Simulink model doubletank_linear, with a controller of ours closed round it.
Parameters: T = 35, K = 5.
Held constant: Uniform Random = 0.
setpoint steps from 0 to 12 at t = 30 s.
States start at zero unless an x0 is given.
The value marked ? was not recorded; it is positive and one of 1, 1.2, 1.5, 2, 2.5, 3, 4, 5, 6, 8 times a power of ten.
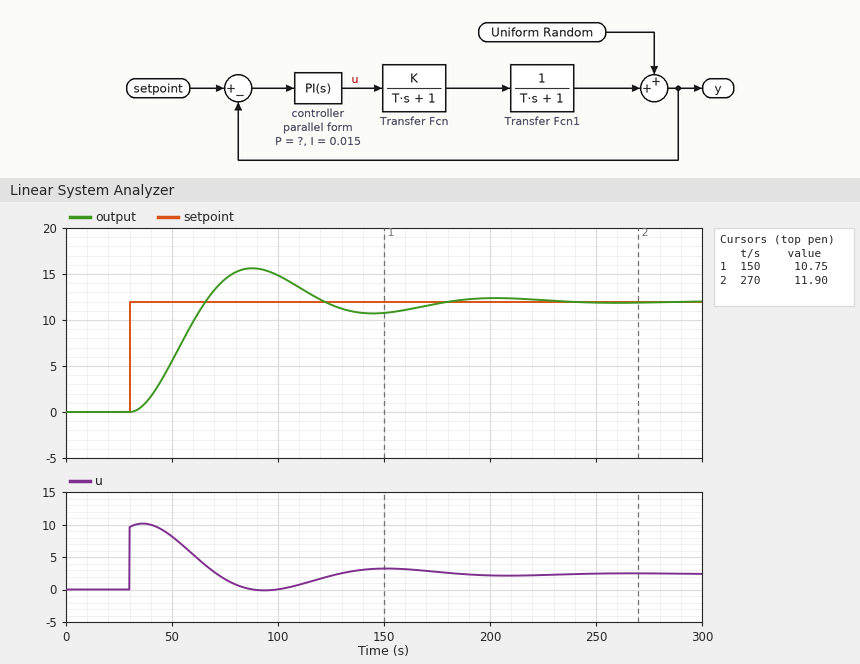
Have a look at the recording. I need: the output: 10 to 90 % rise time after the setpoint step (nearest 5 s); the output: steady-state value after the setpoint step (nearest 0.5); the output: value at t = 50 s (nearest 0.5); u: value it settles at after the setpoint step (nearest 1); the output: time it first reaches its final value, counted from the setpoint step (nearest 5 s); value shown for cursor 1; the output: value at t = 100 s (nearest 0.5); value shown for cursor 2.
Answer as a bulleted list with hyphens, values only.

- 25 s
- 12.0
- 5.5
- 2
- 35 s
- 10.75
- 15.0
- 11.90
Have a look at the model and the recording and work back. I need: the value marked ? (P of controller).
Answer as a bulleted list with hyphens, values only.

- 0.8
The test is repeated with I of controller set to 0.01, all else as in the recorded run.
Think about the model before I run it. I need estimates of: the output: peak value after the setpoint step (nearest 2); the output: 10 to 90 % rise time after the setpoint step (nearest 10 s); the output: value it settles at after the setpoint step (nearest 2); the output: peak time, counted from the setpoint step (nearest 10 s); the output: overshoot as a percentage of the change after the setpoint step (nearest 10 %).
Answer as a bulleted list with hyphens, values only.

- 14
- 30 s
- 12
- 60 s
- 20 %
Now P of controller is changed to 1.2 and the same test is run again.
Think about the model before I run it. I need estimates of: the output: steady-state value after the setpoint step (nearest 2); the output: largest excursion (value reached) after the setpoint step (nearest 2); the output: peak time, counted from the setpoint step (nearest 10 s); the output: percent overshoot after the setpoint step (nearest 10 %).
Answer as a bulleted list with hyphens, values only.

- 12
- 16
- 50 s
- 30 %
